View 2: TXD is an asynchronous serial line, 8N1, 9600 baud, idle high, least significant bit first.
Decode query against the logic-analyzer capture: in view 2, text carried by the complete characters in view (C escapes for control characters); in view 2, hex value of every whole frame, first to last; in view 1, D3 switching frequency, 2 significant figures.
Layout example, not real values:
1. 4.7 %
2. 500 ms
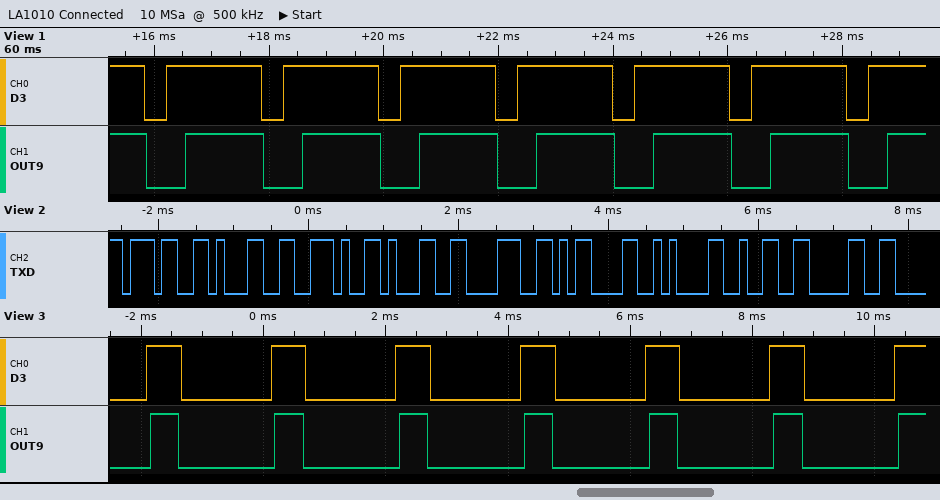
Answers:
1. "71.18\r\n20"
2. 0x37 0x31 0x2E 0x31 0x38 0x0D 0x0A 0x32 0x30
3. 490 Hz
